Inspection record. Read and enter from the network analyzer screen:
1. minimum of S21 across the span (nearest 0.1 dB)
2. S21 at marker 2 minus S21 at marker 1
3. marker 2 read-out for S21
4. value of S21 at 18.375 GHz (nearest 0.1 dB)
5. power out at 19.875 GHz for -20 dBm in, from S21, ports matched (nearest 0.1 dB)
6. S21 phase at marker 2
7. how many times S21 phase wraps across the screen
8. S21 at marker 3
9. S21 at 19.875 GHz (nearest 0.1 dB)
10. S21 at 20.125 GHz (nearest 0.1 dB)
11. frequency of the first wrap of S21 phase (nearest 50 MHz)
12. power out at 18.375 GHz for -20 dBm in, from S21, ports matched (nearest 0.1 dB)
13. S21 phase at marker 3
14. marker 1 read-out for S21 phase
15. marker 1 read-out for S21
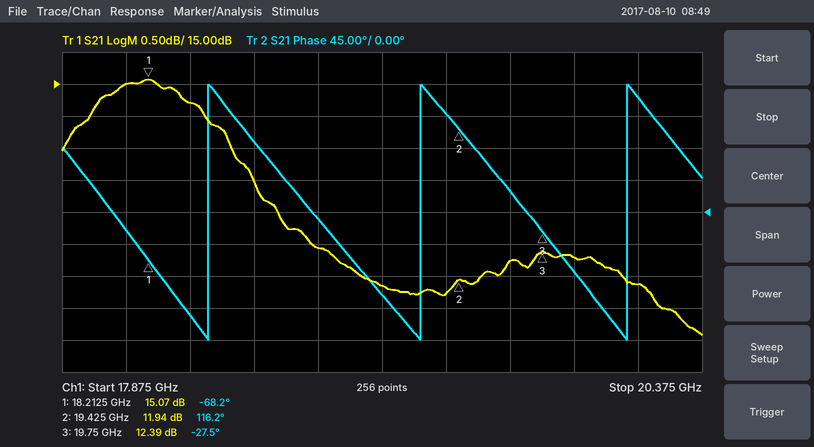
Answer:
11.1 dB
-3.13 dB
11.94 dB
14.7 dB
-7.7 dBm
116.2°
3
12.39 dB
12.3 dB
11.9 dB
18.45 GHz
-5.3 dBm
-27.5°
-68.2°
15.07 dB
